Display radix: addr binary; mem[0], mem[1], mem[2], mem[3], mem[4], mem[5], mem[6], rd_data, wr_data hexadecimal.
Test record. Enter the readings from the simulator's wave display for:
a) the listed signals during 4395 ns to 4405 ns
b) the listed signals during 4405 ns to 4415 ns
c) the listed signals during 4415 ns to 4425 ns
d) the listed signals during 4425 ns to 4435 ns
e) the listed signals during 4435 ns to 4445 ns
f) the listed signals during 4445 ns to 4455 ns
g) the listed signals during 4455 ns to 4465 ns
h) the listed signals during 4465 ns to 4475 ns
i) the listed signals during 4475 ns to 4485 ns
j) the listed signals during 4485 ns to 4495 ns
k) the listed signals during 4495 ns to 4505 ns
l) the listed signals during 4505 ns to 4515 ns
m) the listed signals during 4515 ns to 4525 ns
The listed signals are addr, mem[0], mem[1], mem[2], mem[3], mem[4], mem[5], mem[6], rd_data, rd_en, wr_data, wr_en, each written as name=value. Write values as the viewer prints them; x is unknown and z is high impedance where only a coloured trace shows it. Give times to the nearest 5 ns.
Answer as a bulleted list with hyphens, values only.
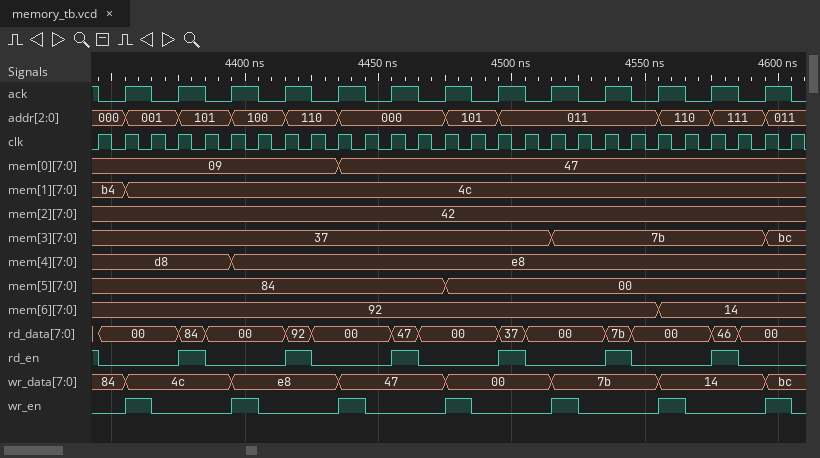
- addr=100, mem[0]=09, mem[1]=4c, mem[2]=42, mem[3]=37, mem[4]=e8, mem[5]=84, mem[6]=92, rd_data=00, rd_en=0, wr_data=e8, wr_en=1
- addr=100, mem[0]=09, mem[1]=4c, mem[2]=42, mem[3]=37, mem[4]=e8, mem[5]=84, mem[6]=92, rd_data=00, rd_en=0, wr_data=e8, wr_en=0
- addr=110, mem[0]=09, mem[1]=4c, mem[2]=42, mem[3]=37, mem[4]=e8, mem[5]=84, mem[6]=92, rd_data=92, rd_en=1, wr_data=e8, wr_en=0
- addr=110, mem[0]=09, mem[1]=4c, mem[2]=42, mem[3]=37, mem[4]=e8, mem[5]=84, mem[6]=92, rd_data=00, rd_en=0, wr_data=e8, wr_en=0
- addr=000, mem[0]=47, mem[1]=4c, mem[2]=42, mem[3]=37, mem[4]=e8, mem[5]=84, mem[6]=92, rd_data=00, rd_en=0, wr_data=47, wr_en=1
- addr=000, mem[0]=47, mem[1]=4c, mem[2]=42, mem[3]=37, mem[4]=e8, mem[5]=84, mem[6]=92, rd_data=00, rd_en=0, wr_data=47, wr_en=0
- addr=000, mem[0]=47, mem[1]=4c, mem[2]=42, mem[3]=37, mem[4]=e8, mem[5]=84, mem[6]=92, rd_data=47, rd_en=1, wr_data=47, wr_en=0
- addr=000, mem[0]=47, mem[1]=4c, mem[2]=42, mem[3]=37, mem[4]=e8, mem[5]=84, mem[6]=92, rd_data=00, rd_en=0, wr_data=47, wr_en=0
- addr=101, mem[0]=47, mem[1]=4c, mem[2]=42, mem[3]=37, mem[4]=e8, mem[5]=00, mem[6]=92, rd_data=00, rd_en=0, wr_data=00, wr_en=1
- addr=101, mem[0]=47, mem[1]=4c, mem[2]=42, mem[3]=37, mem[4]=e8, mem[5]=00, mem[6]=92, rd_data=00, rd_en=0, wr_data=00, wr_en=0
- addr=011, mem[0]=47, mem[1]=4c, mem[2]=42, mem[3]=37, mem[4]=e8, mem[5]=00, mem[6]=92, rd_data=37, rd_en=1, wr_data=00, wr_en=0
- addr=011, mem[0]=47, mem[1]=4c, mem[2]=42, mem[3]=37, mem[4]=e8, mem[5]=00, mem[6]=92, rd_data=00, rd_en=0, wr_data=00, wr_en=0
- addr=011, mem[0]=47, mem[1]=4c, mem[2]=42, mem[3]=7b, mem[4]=e8, mem[5]=00, mem[6]=92, rd_data=00, rd_en=0, wr_data=7b, wr_en=1
